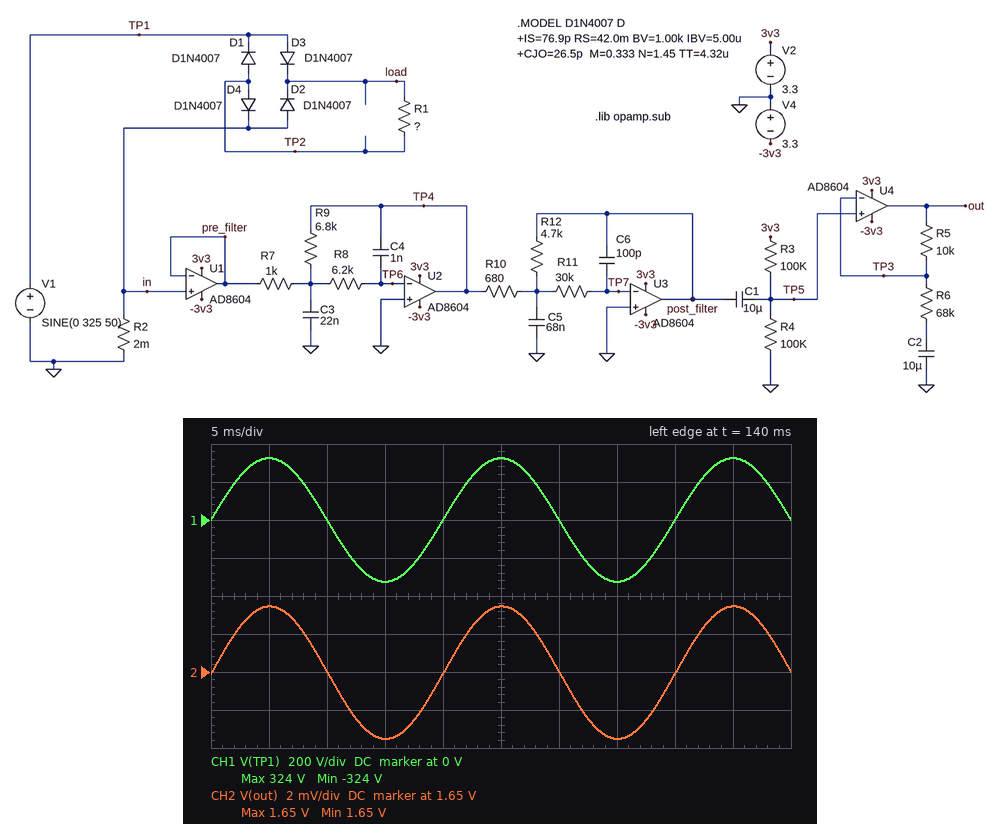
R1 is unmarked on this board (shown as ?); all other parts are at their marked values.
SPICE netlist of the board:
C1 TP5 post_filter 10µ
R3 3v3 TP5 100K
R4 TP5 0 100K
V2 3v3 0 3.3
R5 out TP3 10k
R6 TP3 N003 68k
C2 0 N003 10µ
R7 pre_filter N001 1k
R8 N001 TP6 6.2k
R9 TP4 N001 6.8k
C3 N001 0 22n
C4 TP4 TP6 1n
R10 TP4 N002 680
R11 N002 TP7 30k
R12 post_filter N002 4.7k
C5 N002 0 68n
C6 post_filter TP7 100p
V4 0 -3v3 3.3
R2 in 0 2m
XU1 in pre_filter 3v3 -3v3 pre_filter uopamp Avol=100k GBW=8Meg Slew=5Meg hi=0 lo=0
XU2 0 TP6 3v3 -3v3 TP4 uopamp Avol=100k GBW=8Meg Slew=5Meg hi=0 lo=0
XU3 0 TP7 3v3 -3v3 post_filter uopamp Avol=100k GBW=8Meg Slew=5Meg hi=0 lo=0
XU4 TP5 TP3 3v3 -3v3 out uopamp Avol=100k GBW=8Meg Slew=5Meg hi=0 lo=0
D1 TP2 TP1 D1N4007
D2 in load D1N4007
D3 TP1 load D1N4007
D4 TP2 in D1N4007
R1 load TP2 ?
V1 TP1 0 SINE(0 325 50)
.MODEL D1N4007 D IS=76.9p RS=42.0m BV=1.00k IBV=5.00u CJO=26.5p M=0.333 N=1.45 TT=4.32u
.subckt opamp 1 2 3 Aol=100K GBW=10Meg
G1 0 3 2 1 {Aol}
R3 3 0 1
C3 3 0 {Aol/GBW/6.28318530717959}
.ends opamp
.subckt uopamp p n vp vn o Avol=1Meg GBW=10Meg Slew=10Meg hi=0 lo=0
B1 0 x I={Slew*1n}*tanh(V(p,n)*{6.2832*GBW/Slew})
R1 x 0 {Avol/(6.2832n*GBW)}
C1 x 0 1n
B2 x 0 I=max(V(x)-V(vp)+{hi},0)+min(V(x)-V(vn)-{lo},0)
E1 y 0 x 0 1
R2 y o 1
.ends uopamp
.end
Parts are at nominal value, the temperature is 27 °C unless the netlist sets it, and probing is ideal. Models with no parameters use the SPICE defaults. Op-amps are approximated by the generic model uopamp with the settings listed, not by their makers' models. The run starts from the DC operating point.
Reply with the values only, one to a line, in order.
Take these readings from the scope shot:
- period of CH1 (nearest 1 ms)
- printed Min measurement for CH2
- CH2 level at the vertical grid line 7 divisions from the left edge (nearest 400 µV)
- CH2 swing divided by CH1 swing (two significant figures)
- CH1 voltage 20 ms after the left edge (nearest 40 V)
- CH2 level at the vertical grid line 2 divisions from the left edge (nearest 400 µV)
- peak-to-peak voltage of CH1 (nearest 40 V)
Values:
20 ms
1.65 V
1.6464 V
0.000011
0 V
1.6500 V
640 V
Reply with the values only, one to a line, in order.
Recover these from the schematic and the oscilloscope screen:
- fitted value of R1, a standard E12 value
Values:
10 kΩ
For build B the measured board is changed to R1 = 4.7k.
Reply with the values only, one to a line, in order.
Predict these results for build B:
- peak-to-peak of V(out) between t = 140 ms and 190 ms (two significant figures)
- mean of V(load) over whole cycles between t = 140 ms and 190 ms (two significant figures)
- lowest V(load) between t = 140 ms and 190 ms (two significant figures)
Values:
15 mV
100 V
-780 mV
